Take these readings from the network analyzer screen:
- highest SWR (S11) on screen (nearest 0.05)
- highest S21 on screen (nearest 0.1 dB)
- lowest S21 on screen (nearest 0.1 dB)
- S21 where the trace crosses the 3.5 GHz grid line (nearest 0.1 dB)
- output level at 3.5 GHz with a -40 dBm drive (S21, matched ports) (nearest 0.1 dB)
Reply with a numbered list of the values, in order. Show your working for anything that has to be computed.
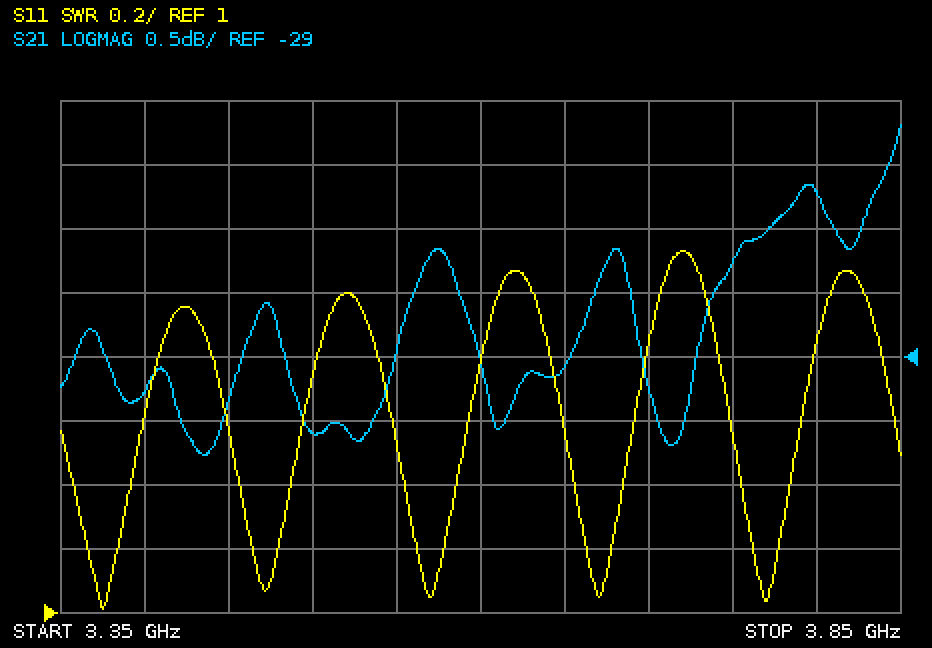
1. 2.15
2. -27.2 dB
3. -29.8 dB
4. -29.6 dB
5. -40 dBm + (-29.6 dB) = -69.6 dBm
